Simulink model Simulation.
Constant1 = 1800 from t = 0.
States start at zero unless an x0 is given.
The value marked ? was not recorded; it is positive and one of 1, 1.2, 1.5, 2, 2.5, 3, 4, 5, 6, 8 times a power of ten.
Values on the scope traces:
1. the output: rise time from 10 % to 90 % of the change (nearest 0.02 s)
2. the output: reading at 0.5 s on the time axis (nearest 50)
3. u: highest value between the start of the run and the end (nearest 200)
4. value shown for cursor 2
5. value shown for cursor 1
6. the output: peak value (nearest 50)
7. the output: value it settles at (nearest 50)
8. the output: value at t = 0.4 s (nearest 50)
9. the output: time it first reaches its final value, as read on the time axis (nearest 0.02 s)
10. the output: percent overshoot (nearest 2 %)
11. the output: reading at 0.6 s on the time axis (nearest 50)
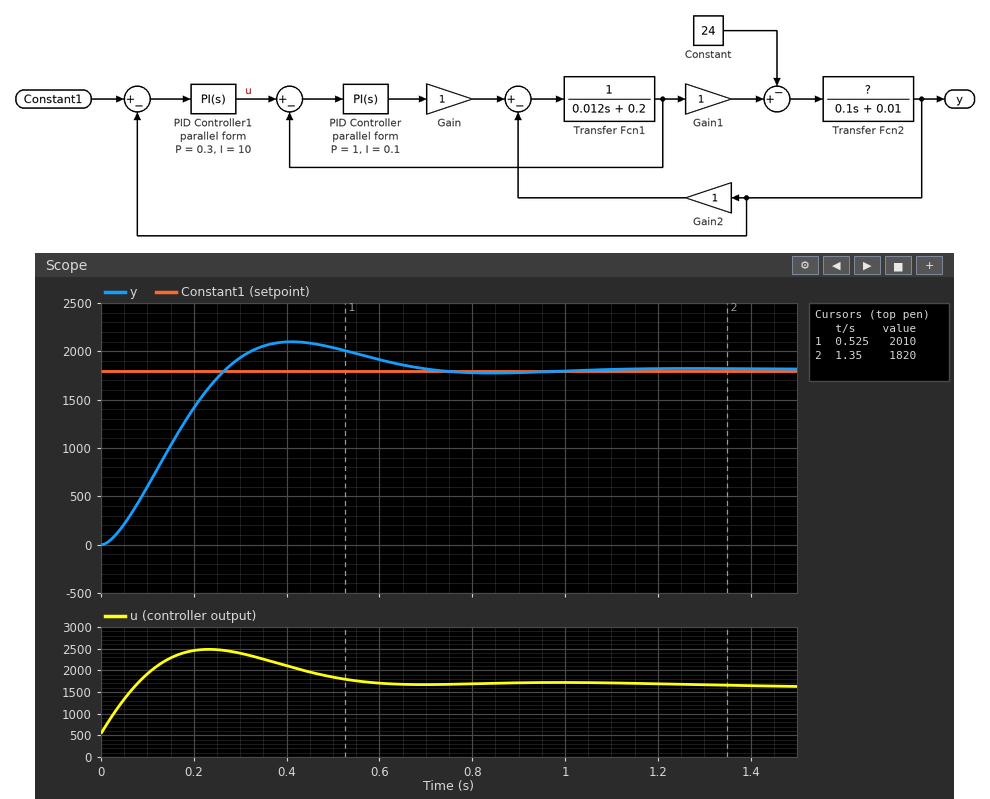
0.18 s
2050
2400
1820
2010
2100
1800
2100
0.26 s
16 %
1900
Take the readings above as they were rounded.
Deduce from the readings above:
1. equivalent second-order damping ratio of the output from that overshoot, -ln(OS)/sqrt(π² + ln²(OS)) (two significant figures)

0.50
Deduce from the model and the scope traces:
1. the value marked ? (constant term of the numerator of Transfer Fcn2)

0.8
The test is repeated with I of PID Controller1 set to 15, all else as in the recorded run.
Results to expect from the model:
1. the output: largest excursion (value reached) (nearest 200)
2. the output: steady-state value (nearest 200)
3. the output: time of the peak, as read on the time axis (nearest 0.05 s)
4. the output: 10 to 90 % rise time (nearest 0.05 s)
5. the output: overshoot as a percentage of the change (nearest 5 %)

2200
1800
0.30 s
0.15 s
25 %
